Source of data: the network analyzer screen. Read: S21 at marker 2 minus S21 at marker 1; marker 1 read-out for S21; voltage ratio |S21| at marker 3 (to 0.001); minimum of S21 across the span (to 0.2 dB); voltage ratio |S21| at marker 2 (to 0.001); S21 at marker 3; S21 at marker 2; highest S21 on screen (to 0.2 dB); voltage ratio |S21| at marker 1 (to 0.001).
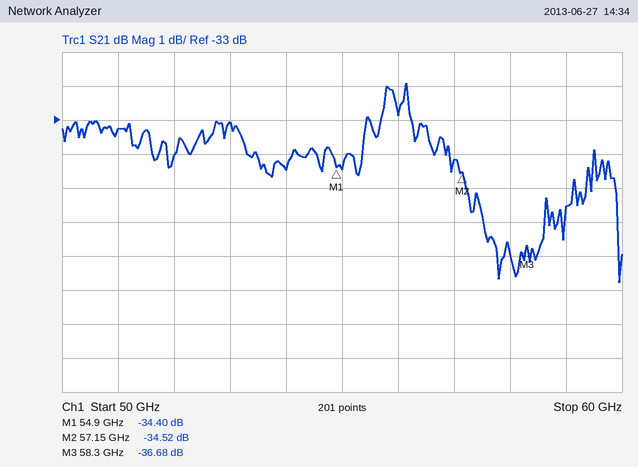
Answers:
-0.12 dB
-34.40 dB
0.015
-37.8 dB
0.019
-36.68 dB
-34.52 dB
-32.0 dB
0.019
